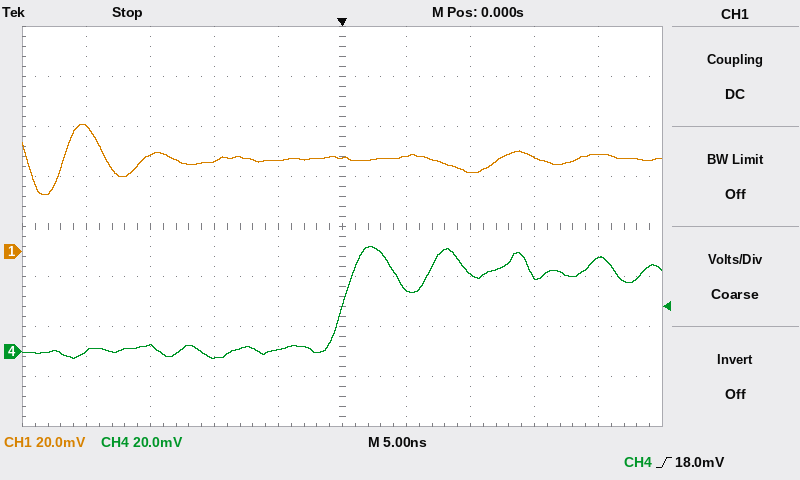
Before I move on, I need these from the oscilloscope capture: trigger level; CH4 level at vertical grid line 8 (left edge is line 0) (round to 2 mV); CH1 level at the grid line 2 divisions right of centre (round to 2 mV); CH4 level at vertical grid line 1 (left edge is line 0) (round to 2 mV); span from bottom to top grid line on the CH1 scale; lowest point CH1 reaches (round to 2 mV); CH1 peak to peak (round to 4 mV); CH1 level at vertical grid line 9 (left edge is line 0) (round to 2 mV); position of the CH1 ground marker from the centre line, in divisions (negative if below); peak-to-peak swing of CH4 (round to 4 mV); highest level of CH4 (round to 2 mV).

18.0 mV
30 mV
32 mV
0 mV
160 mV
22 mV
28 mV
38 mV
-0.5 div
44 mV
42 mV
